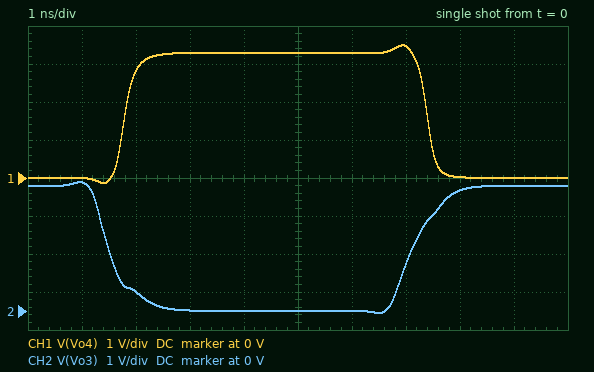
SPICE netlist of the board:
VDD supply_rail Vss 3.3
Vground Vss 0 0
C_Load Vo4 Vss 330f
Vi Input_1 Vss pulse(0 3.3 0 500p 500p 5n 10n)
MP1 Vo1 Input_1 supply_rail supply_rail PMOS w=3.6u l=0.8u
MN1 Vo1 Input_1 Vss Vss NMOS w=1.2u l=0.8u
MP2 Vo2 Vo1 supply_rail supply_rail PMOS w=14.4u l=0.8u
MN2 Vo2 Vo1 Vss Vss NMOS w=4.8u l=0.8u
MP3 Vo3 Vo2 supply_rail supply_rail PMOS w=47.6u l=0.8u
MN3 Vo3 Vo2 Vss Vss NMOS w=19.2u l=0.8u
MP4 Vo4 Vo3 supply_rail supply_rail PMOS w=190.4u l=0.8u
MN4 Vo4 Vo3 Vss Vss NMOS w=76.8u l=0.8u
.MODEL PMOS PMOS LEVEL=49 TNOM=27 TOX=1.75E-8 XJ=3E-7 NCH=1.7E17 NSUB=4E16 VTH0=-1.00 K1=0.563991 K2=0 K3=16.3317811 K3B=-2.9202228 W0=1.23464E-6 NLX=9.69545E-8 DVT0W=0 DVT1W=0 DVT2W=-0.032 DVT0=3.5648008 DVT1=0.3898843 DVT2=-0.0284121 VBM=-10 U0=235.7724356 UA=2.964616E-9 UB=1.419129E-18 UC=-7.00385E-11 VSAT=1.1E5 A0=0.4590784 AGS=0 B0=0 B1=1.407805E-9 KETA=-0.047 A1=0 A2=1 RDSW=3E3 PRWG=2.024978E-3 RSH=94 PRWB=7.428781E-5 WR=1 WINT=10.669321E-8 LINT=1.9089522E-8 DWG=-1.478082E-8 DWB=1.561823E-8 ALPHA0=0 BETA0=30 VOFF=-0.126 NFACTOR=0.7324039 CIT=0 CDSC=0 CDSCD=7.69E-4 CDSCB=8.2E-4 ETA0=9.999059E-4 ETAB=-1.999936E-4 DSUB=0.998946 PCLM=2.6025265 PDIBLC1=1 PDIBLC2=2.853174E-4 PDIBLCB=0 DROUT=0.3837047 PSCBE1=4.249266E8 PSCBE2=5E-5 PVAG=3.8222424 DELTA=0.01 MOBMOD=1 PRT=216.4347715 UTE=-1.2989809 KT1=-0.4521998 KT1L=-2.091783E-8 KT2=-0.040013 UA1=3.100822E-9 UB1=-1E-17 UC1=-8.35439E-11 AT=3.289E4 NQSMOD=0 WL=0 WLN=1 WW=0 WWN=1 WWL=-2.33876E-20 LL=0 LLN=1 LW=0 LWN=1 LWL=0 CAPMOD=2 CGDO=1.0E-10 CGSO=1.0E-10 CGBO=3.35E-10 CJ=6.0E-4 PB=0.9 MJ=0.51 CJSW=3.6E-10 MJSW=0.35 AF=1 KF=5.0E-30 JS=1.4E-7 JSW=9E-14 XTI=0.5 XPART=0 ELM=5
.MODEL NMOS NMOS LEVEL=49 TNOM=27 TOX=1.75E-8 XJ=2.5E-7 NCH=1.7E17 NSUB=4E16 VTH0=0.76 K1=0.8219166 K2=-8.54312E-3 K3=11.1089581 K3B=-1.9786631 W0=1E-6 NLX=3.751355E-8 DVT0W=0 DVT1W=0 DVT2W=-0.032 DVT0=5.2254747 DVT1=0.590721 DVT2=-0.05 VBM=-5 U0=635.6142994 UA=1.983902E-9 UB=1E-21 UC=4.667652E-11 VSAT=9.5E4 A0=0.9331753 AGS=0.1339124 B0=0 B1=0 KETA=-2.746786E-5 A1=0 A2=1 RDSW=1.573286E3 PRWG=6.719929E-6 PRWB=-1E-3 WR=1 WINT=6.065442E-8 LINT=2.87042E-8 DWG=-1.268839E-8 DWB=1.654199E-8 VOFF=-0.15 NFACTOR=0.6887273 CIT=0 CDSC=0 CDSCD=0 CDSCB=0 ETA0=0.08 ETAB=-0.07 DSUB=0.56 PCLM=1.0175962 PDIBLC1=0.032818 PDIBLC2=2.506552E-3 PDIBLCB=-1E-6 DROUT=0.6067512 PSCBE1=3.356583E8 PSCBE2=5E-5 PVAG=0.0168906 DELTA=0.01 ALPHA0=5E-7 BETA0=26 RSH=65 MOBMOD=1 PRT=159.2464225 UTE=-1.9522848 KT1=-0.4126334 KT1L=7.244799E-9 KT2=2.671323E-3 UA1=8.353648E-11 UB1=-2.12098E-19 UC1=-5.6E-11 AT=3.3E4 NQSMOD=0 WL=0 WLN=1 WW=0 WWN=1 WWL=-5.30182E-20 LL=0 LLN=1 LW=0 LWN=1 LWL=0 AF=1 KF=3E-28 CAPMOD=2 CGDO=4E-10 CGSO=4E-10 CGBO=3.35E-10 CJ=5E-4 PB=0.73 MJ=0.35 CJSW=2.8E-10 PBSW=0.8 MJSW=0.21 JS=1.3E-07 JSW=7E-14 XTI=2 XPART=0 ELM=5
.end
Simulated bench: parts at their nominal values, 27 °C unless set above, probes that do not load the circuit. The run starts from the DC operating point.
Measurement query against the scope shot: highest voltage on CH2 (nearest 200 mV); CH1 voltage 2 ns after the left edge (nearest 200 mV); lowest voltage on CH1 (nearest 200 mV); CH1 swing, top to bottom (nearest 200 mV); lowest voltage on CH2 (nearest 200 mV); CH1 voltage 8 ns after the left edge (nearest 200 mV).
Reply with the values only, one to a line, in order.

3.4 V
2.8 V
-200 mV
3.6 V
0 V
0 V
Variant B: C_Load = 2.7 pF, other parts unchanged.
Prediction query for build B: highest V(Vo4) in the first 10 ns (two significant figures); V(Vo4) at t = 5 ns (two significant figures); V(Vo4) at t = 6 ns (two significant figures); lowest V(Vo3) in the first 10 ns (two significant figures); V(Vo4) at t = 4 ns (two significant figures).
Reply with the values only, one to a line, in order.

3.4 V
3.2 V
3.3 V
-53 mV
3.0 V
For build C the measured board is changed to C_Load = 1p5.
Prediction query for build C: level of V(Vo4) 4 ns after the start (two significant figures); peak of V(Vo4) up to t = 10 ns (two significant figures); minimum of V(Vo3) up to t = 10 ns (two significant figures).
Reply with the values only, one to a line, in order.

3.3 V
3.4 V
-55 mV
